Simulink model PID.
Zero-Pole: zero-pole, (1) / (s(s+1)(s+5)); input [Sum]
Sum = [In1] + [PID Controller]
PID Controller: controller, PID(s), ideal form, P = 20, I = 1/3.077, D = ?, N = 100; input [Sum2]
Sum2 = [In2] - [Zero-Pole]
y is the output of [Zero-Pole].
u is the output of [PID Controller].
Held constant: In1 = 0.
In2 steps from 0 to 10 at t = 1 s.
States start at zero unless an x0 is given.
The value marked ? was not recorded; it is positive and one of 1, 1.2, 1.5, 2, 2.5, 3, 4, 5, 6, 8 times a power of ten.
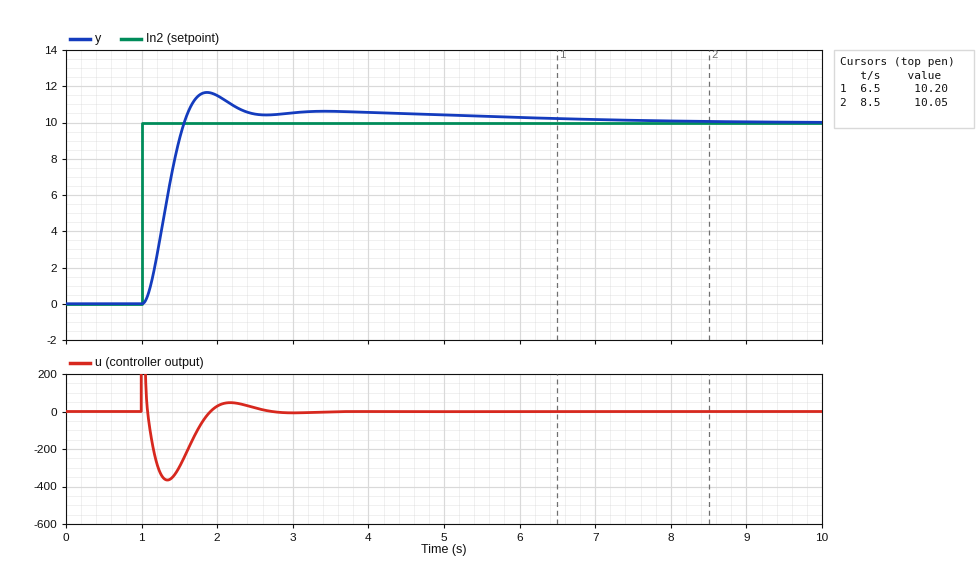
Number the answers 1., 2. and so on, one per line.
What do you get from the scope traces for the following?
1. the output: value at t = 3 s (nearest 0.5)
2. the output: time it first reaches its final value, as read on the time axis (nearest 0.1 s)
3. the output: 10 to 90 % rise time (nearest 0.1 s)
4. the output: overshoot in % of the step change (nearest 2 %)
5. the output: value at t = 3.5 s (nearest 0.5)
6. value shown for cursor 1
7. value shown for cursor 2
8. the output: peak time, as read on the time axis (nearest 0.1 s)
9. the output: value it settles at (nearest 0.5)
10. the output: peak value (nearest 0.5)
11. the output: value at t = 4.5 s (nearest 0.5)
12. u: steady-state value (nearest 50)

1. 10.5
2. 1.6 s
3. 0.4 s
4. 16 %
5. 10.5
6. 10.20
7. 10.05
8. 1.9 s
9. 10.0
10. 11.5
11. 10.5
12. 0
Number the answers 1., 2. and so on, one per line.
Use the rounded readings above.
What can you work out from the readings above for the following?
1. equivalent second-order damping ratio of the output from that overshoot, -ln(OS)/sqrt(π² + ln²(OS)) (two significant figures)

1. 0.50
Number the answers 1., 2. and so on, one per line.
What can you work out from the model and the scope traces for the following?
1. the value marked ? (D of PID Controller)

1. 1
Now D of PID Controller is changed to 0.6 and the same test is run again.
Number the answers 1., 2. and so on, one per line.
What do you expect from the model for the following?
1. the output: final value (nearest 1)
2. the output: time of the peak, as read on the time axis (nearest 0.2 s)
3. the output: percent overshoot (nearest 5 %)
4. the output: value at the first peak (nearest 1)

1. 10
2. 2.2 s
3. 25 %
4. 13
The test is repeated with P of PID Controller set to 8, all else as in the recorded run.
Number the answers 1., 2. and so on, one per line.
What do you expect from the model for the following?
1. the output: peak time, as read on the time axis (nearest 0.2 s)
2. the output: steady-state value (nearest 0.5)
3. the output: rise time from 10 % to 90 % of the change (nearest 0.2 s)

1. 4.2 s
2. 10.0
3. 0.8 s
